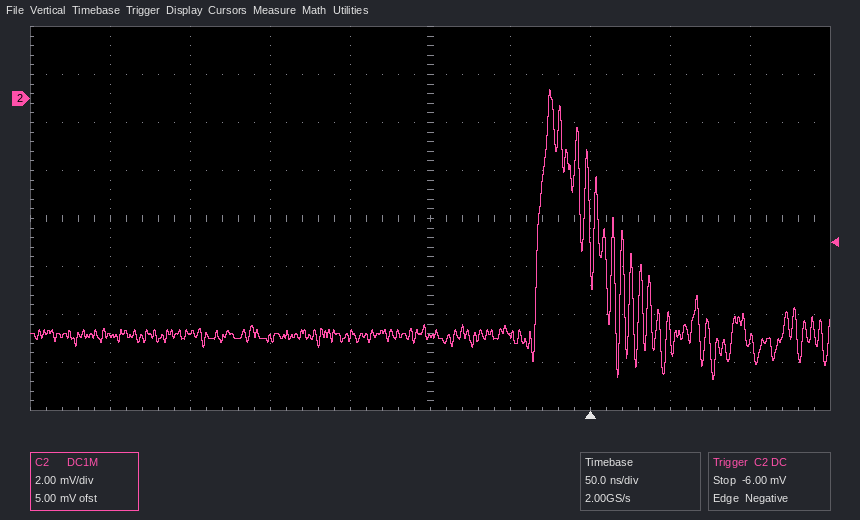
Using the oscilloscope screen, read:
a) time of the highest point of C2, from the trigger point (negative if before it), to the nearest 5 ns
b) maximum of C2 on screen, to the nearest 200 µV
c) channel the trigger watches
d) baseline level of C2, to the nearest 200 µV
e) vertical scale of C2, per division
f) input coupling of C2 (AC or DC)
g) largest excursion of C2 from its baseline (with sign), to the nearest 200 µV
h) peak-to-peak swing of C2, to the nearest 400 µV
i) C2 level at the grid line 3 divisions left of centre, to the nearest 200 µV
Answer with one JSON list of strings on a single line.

["-25 ns", "400 µV", "C2", "-9.8 mV", "2 mV", "DC", "+10.2 mV", "12.0 mV", "-9.8 mV"]
